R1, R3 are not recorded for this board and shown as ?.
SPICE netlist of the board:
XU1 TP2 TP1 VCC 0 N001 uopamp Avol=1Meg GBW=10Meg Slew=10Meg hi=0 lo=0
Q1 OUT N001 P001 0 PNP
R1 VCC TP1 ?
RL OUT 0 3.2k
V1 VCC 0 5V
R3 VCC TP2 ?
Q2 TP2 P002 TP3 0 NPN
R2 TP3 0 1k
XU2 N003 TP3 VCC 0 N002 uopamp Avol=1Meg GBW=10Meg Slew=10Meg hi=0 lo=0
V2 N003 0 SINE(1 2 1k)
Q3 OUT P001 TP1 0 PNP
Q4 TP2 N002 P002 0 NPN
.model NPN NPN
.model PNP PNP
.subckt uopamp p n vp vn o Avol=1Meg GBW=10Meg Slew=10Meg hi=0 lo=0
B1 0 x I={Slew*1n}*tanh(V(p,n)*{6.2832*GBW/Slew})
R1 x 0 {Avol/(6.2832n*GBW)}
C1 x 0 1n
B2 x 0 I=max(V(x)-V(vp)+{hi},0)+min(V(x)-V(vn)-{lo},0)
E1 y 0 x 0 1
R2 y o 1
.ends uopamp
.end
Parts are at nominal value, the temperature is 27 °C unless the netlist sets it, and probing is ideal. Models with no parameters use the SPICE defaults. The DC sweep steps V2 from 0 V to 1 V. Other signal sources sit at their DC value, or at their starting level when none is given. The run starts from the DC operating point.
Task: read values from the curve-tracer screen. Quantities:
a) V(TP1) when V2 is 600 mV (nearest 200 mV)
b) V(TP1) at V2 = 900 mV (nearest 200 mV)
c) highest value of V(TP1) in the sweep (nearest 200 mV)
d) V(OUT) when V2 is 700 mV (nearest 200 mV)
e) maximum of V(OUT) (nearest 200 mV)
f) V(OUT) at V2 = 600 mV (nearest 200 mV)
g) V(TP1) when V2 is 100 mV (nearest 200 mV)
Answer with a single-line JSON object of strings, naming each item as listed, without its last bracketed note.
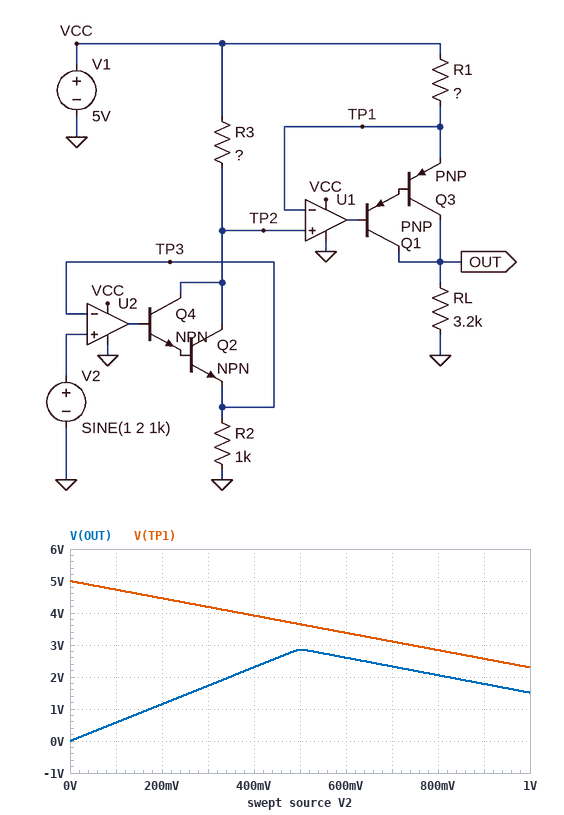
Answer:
{"V(TP1) when V2 is 600 mV": "3.4 V", "V(TP1) at V2 = 900 mV": "2.6 V", "highest value of V(TP1) in the sweep": "5.0 V", "V(OUT) when V2 is 700 mV": "2.4 V", "maximum of V(OUT)": "2.8 V", "V(OUT) at V2 = 600 mV": "2.6 V", "V(TP1) when V2 is 100 mV": "4.8 V"}
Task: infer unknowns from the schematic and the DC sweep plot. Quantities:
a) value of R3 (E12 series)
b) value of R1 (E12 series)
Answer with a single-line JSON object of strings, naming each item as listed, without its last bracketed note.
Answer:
{"value of R3": "2.7 kΩ", "value of R1": "1.5 kΩ"}
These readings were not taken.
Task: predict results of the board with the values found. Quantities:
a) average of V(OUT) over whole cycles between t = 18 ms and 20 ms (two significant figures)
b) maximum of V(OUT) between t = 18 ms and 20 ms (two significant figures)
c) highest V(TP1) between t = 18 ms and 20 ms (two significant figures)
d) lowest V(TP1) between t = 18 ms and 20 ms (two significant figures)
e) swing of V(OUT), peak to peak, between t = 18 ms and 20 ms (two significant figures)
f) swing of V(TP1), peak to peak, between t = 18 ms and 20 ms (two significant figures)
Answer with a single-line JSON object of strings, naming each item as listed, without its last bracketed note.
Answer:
{"average of V(OUT) over whole cycles between t = 18 ms and 20 ms": "1.4 V", "maximum of V(OUT) between t = 18 ms and 20 ms": "2.9 V", "highest V(TP1) between t = 18 ms and 20 ms": "5.0 V", "lowest V(TP1) between t = 18 ms and 20 ms": "1.9 V", "swing of V(OUT), peak to peak, between t = 18 ms and 20 ms": "2.9 V", "swing of V(TP1), peak to peak, between t = 18 ms and 20 ms": "3.1 V"}
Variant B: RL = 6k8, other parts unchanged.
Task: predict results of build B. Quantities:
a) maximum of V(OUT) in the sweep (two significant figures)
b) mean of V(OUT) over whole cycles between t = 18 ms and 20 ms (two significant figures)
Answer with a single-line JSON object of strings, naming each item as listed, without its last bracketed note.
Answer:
{"maximum of V(OUT) in the sweep": "3.5 V", "mean of V(OUT) over whole cycles between t = 18 ms and 20 ms": "1.5 V"}
